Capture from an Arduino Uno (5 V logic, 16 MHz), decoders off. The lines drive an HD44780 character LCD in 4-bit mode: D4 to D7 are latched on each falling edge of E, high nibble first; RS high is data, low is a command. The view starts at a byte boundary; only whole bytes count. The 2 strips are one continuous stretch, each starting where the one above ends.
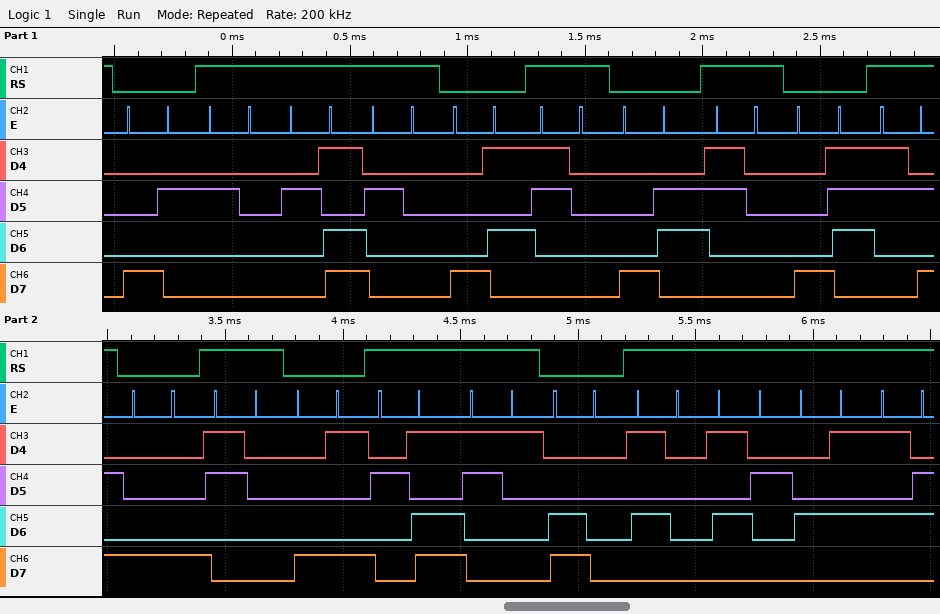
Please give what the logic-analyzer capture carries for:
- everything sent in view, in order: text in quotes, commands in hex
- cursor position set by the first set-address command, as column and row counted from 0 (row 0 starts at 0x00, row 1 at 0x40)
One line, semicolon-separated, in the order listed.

0x82 " - " 0x85 "0" 0x86 "0" 0x87 ":" 0x88 "0" 0x89 "-1" 0xC0 "PREV"; column 2, row 0
